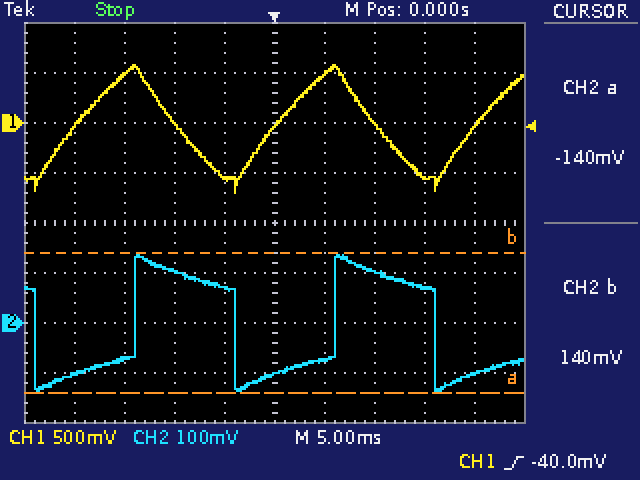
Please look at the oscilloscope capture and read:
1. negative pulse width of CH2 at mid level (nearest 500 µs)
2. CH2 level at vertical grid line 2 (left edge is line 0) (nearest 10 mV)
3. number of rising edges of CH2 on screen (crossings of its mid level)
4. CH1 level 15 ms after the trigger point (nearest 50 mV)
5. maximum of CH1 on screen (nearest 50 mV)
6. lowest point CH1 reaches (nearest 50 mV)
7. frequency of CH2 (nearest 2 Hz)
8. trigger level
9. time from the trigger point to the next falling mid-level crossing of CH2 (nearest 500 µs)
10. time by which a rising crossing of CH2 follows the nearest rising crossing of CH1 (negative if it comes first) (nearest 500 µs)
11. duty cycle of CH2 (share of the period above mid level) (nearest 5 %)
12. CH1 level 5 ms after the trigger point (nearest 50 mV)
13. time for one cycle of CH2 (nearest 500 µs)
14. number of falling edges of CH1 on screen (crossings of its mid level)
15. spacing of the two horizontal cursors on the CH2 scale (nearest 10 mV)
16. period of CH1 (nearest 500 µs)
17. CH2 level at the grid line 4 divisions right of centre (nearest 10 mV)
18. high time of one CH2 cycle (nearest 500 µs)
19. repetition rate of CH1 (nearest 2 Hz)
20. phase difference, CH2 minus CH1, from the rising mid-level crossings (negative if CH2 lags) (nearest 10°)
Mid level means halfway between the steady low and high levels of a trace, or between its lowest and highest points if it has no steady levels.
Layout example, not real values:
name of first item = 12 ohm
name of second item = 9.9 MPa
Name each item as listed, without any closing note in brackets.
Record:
negative pulse width of CH2 at mid level = 10.0 ms
CH2 level at vertical grid line 2 (left edge is line 0) = -70 mV
number of rising edges of CH2 on screen = 2
CH1 level 15 ms after the trigger point = -550 mV
maximum of CH1 on screen = 600 mV
lowest point CH1 reaches = -700 mV
frequency of CH2 = 50 Hz
trigger level = -40.0 mV
time from the trigger point to the next falling mid-level crossing of CH2 = 16.0 ms
time by which a rising crossing of CH2 follows the nearest rising crossing of CH1 (negative if it comes first) = +6.0 ms
duty cycle of CH2 (share of the period above mid level) = 50 %
CH1 level 5 ms after the trigger point = 500 mV
time for one cycle of CH2 = 20.0 ms
number of falling edges of CH1 on screen = 2
spacing of the two horizontal cursors on the CH2 scale = 280 mV
period of CH1 = 20.0 ms
CH2 level at the grid line 4 divisions right of centre = -100 mV
high time of one CH2 cycle = 10.0 ms
repetition rate of CH1 = 50 Hz
phase difference, CH2 minus CH1, from the rising mid-level crossings (negative if CH2 lags) = -110°
